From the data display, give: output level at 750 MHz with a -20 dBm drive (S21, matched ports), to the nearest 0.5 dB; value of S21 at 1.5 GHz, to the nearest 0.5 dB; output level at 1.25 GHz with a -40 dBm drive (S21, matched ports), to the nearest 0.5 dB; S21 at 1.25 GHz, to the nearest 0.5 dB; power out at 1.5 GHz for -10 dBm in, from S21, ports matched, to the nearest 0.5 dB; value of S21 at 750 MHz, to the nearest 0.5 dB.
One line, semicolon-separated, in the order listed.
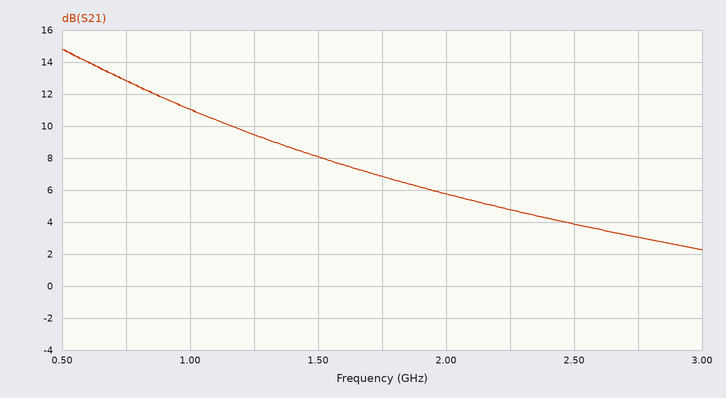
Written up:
-7.0 dBm; 8.0 dB; -30.5 dBm; 9.5 dB; -2.0 dBm; 13.0 dB
